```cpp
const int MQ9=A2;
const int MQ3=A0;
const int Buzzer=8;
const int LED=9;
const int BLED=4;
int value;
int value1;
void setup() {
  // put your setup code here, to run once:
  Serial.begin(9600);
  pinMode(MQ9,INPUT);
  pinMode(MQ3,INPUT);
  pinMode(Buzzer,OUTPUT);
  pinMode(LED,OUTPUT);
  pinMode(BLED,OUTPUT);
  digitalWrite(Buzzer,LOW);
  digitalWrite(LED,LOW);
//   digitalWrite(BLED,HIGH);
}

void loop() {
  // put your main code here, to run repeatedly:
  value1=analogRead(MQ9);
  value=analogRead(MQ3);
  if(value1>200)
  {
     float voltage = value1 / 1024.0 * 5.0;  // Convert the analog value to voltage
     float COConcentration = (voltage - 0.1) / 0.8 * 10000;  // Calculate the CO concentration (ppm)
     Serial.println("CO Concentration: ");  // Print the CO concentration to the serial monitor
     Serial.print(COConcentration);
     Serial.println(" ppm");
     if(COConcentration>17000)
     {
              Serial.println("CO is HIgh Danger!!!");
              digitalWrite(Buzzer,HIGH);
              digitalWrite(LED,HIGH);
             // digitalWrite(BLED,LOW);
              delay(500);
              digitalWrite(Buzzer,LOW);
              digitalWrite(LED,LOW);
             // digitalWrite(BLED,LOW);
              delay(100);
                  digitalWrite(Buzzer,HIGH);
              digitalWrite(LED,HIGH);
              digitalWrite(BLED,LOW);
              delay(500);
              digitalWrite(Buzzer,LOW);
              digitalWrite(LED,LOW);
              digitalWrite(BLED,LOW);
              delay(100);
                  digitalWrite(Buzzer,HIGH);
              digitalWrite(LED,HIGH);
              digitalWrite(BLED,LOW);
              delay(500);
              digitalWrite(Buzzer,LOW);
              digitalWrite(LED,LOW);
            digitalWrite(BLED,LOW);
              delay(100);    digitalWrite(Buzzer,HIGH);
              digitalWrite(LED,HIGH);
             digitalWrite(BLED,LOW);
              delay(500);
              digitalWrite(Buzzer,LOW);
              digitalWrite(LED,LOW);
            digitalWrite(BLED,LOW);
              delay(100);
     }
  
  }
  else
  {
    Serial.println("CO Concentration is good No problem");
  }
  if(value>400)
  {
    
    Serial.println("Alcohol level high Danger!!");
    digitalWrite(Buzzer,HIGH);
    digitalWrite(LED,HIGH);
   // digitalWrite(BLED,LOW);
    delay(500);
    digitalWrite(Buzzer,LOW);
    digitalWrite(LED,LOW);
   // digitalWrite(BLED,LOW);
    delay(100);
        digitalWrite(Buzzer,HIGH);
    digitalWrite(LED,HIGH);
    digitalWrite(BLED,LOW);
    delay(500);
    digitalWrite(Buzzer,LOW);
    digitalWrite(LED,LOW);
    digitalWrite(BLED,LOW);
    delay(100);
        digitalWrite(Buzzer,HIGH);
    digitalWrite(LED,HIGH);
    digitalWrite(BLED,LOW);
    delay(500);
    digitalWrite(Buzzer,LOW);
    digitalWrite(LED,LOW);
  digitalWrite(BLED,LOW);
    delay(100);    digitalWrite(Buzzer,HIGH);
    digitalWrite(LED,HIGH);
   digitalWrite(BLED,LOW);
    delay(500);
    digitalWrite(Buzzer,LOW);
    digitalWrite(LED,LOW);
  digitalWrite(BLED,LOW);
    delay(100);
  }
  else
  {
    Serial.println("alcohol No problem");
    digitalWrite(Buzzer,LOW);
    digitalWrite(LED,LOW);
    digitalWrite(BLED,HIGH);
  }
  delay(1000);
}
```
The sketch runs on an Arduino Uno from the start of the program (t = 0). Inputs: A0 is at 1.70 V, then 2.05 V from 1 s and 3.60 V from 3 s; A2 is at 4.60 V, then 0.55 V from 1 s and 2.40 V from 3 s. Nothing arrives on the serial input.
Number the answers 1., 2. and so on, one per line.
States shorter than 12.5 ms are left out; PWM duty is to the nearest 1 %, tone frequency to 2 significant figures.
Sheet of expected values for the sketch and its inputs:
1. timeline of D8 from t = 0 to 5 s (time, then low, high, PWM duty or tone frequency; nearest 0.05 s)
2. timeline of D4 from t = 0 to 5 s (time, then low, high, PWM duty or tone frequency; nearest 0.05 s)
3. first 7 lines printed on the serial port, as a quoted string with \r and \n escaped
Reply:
1. 0 s high; 0.5 s low; 0.6 s high; 1.1 s low; 1.2 s high; 1.7 s low; 1.8 s high; 2.3 s low; 3.4 s high; 3.9 s low; 4 s high; 4.5 s low; 4.6 s high
2. 0 s low; 2.4 s high; 4 s low
3. "CO Concentration: \r\n56245.12 ppm\r\nCO is HIgh Danger!!!\r\nalcohol No problem\r\nCO Concentration: \r\n28718.26 ppm\r\nCO is HIgh Danger!!!\r\n"
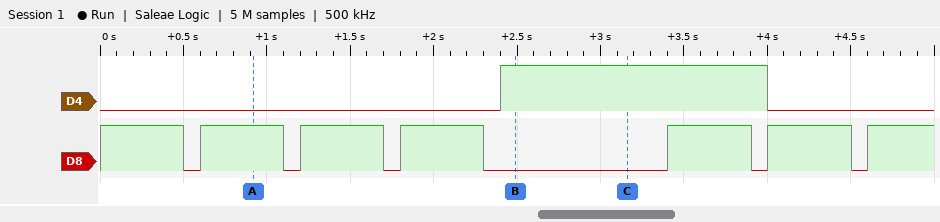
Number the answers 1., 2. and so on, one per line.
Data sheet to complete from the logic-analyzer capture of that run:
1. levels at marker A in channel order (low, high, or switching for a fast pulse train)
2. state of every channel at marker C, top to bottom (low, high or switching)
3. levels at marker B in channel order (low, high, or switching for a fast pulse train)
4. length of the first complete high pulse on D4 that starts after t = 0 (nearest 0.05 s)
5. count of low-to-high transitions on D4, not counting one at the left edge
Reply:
1. D4 low, D8 high
2. D4 high, D8 low
3. D4 high, D8 low
4. 1.60 s
5. 1
